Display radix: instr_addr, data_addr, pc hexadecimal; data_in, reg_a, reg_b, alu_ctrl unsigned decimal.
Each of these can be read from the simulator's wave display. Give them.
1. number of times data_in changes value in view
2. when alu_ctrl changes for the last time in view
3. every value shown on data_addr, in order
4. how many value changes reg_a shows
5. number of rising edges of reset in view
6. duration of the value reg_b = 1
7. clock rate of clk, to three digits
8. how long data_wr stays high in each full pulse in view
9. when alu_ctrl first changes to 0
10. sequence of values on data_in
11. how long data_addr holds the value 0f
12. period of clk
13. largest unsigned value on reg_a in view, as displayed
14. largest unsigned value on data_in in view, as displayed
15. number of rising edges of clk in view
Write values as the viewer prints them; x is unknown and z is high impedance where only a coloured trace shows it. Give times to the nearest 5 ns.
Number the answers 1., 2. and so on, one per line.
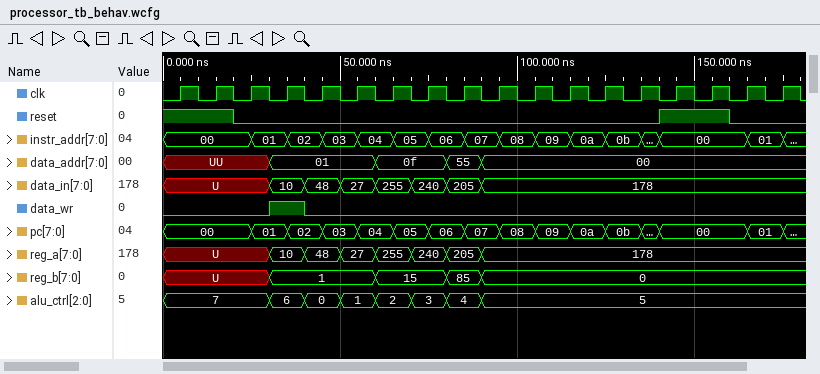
1. 7
2. 90 ns
3. UU, 01, 0f, 55, 00
4. 7
5. 1
6. 30 ns
7. 100 MHz
8. 10 ns
9. 40 ns
10. U, 10, 48, 27, 255, 240, 205, 178
11. 20 ns
12. 10 ns
13. 255
14. 255
15. 18
